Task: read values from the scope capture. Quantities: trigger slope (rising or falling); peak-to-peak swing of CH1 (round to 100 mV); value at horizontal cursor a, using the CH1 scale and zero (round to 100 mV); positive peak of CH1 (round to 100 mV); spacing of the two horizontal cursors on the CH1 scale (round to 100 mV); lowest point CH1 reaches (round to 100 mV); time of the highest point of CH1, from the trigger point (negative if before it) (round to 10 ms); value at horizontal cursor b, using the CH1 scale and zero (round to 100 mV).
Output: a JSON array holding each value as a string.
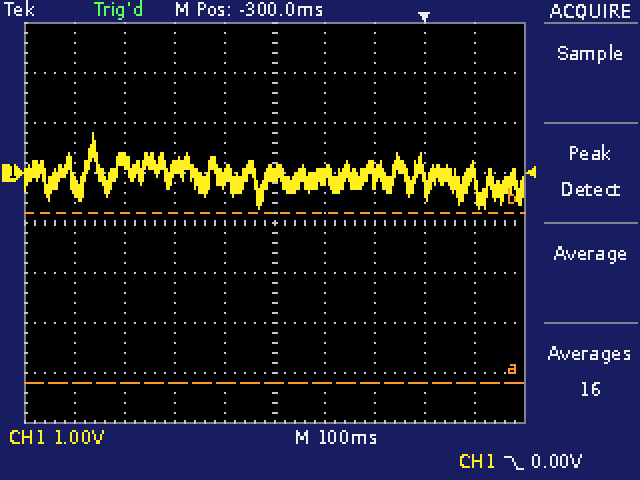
["falling", "1.5 V", "-4.2 V", "800 mV", "3.4 V", "-700 mV", "-660 ms", "-800 mV"]
